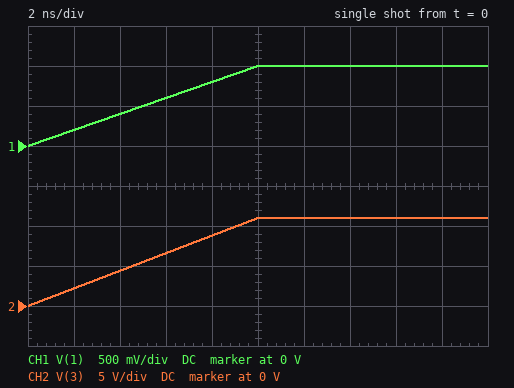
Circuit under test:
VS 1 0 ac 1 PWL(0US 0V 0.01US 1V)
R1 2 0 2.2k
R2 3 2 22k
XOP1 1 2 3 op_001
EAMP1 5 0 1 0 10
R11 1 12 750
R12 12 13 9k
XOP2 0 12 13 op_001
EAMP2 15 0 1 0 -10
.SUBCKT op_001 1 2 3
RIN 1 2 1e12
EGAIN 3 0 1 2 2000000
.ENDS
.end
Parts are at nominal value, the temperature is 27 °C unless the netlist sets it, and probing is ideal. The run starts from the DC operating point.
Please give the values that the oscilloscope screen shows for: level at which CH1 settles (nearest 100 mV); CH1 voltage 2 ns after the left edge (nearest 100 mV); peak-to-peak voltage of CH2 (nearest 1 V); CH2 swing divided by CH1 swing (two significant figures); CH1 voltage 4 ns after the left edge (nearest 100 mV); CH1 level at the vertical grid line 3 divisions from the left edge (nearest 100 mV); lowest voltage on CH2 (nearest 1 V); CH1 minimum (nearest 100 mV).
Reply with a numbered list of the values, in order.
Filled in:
1. 1.0 V
2. 200 mV
3. 11 V
4. 11
5. 400 mV
6. 600 mV
7. 0 V
8. 0 V
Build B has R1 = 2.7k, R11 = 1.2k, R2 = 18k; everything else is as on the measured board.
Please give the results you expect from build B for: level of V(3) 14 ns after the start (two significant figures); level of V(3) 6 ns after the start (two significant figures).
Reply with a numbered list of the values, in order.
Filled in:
1. 7.7 V
2. 4.6 V
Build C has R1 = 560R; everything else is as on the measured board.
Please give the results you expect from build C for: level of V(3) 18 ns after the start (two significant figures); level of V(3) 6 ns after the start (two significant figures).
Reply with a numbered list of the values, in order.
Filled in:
1. 40 V
2. 24 V
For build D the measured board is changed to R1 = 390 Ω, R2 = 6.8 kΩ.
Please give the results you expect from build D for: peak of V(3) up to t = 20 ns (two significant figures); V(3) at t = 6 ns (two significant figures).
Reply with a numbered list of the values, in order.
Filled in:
1. 18 V
2. 11 V
